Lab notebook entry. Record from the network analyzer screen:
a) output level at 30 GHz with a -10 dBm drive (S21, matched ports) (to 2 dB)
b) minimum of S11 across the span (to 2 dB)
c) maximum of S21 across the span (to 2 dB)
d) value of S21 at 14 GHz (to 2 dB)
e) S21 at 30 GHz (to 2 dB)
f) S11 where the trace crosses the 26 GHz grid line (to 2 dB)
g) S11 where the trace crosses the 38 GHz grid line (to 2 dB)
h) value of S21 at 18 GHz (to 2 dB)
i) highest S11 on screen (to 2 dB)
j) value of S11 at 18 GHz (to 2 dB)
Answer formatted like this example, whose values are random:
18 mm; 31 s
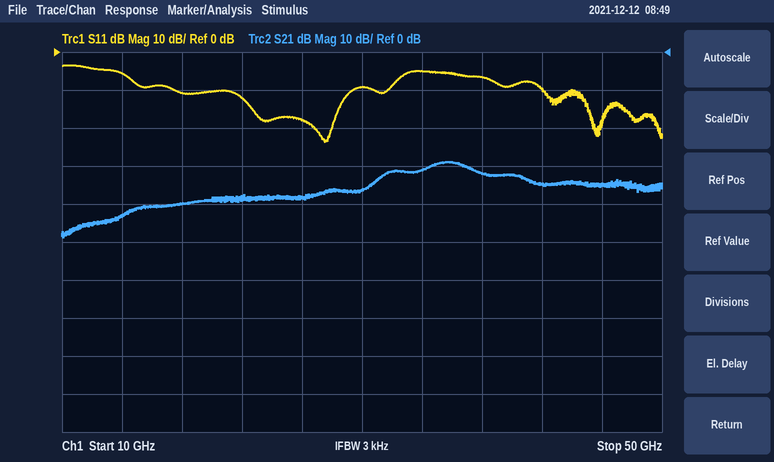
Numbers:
-46 dBm; -24 dB; -28 dB; -44 dB; -36 dB; -18 dB; -6 dB; -40 dB; -4 dB; -10 dB
